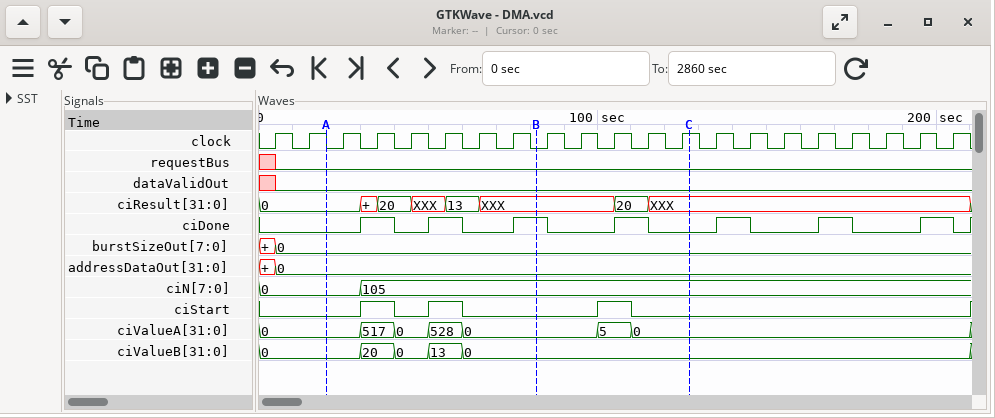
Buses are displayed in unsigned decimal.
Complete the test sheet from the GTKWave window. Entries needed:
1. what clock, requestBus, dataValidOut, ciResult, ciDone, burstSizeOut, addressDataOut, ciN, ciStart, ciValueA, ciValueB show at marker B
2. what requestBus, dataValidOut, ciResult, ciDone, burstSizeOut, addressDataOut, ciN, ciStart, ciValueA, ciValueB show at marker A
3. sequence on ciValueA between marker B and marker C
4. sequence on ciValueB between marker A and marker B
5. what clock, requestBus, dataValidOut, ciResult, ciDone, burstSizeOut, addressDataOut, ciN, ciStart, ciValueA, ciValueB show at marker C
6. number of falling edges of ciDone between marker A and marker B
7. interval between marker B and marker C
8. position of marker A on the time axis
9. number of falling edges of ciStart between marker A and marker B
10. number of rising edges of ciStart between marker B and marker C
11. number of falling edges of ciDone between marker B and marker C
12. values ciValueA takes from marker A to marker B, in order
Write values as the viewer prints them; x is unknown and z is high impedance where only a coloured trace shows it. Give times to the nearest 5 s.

clock=0, requestBus=0, dataValidOut=0, ciResult=XXX, ciDone=1, burstSizeOut=0, addressDataOut=0, ciN=105, ciStart=0, ciValueA=0, ciValueB=0
requestBus=0, dataValidOut=0, ciResult=0, ciDone=0, burstSizeOut=0, addressDataOut=0, ciN=0, ciStart=0, ciValueA=0, ciValueB=0
0, 5, 0
0, 20, 0, 13, 0
clock=1, requestBus=0, dataValidOut=0, ciResult=XXX, ciDone=0, burstSizeOut=0, addressDataOut=0, ciN=105, ciStart=0, ciValueA=0, ciValueB=0
2
45 s
20 s
2
1
2
0, 517, 0, 528, 0
